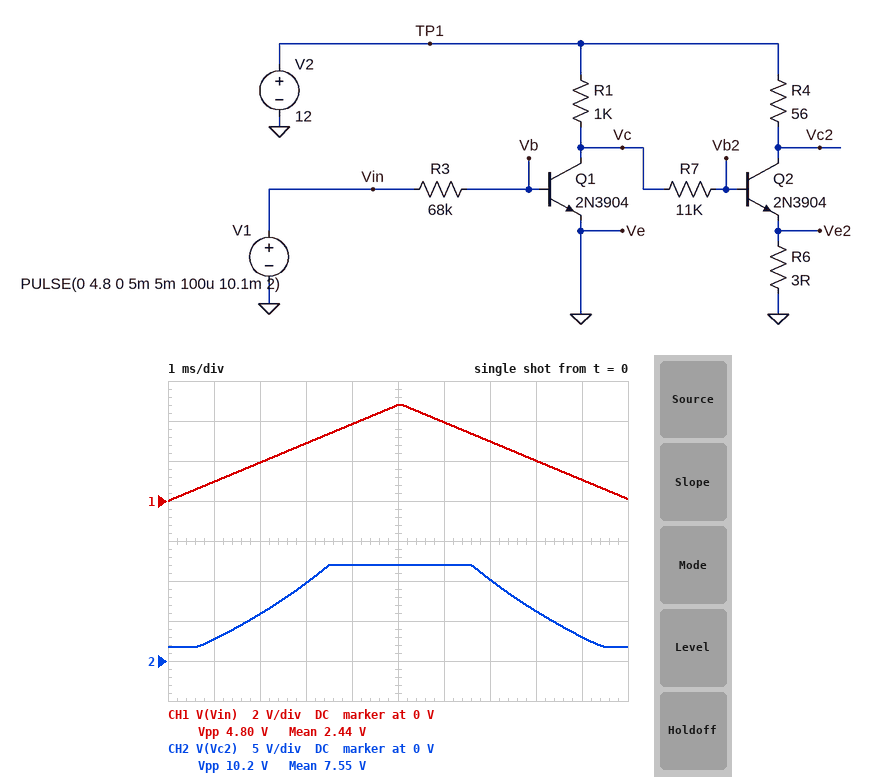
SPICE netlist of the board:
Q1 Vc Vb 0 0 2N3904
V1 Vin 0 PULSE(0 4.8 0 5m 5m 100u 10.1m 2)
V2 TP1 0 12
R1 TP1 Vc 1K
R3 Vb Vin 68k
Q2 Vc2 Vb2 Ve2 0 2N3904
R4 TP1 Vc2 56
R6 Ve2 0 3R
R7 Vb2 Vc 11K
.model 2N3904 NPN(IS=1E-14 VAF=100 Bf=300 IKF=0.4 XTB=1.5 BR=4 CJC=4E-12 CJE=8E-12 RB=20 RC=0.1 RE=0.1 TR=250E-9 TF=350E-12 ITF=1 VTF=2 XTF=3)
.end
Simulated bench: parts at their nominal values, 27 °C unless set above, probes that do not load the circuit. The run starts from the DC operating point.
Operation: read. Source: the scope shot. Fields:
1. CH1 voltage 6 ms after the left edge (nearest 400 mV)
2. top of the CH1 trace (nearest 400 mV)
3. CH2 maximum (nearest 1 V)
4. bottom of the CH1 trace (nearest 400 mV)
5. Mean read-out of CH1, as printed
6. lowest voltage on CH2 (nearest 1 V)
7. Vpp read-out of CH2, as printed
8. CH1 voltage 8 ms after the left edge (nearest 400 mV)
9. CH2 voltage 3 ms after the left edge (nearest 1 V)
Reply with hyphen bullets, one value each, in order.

- 4.0 V
- 4.8 V
- 12 V
- 0 V
- 2.44 V
- 2 V
- 10.2 V
- 2.0 V
- 10 V
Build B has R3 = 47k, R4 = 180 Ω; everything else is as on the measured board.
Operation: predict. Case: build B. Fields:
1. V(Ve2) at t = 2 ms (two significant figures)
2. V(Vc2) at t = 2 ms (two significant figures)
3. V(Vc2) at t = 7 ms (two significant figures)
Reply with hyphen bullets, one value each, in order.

- 190 mV
- 390 mV
- 12 V
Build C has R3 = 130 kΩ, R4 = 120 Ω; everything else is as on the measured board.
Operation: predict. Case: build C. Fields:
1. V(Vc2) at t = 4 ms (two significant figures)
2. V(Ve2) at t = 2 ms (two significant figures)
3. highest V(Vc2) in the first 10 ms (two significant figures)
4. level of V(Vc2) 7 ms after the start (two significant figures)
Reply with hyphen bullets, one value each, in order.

- 2.7 V
- 290 mV
- 7.0 V
- 470 mV
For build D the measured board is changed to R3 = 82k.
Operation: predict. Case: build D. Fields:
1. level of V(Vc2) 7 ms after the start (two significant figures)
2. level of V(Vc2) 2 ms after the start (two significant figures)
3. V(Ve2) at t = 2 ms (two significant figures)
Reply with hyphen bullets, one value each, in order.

- 8.5 V
- 5.1 V
- 370 mV
